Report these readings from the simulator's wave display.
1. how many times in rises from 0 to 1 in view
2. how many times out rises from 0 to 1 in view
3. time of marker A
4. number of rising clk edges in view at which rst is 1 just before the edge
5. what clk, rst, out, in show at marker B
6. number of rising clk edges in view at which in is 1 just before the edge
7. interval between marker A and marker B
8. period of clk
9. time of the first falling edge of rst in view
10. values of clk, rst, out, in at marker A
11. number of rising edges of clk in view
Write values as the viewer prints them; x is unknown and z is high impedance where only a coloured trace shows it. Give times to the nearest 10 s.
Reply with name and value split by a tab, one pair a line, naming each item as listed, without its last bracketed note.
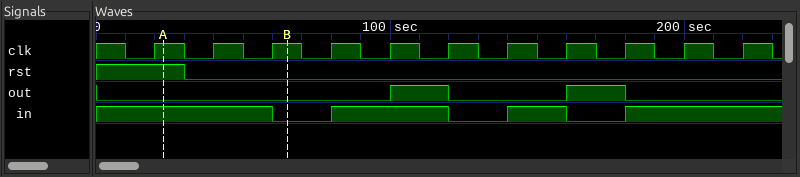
how many times in rises from 0 to 1 in view	3
how many times out rises from 0 to 1 in view	2
time of marker A	20 s
number of rising clk edges in view at which rst is 1 just before the edge	1
what clk, rst, out, in show at marker B	clk=1, rst=0, out=0, in=0
number of rising clk edges in view at which in is 1 just before the edge	8
interval between marker A and marker B	40 s
period of clk	20 s
time of the first falling edge of rst in view	30 s
values of clk, rst, out, in at marker A	clk=1, rst=1, out=0, in=1
number of rising edges of clk in view	11
